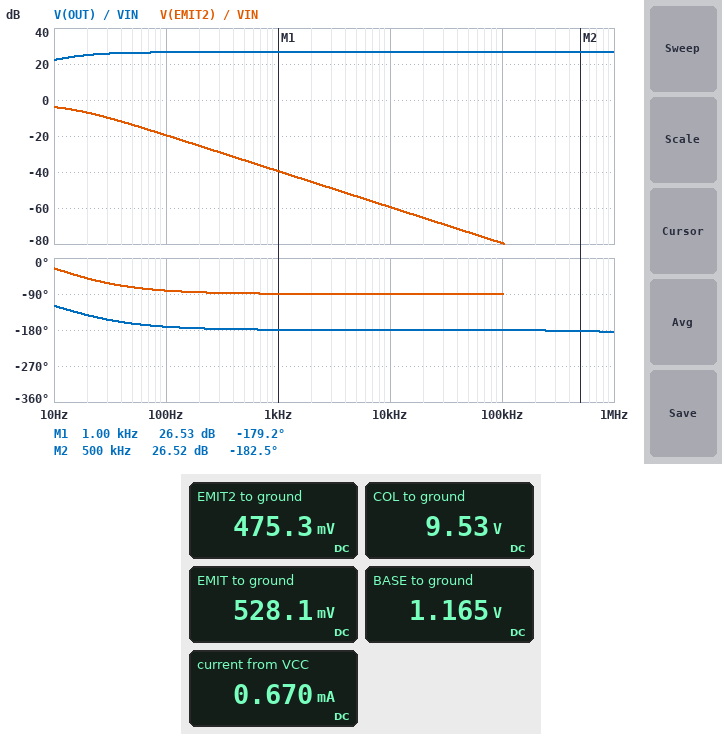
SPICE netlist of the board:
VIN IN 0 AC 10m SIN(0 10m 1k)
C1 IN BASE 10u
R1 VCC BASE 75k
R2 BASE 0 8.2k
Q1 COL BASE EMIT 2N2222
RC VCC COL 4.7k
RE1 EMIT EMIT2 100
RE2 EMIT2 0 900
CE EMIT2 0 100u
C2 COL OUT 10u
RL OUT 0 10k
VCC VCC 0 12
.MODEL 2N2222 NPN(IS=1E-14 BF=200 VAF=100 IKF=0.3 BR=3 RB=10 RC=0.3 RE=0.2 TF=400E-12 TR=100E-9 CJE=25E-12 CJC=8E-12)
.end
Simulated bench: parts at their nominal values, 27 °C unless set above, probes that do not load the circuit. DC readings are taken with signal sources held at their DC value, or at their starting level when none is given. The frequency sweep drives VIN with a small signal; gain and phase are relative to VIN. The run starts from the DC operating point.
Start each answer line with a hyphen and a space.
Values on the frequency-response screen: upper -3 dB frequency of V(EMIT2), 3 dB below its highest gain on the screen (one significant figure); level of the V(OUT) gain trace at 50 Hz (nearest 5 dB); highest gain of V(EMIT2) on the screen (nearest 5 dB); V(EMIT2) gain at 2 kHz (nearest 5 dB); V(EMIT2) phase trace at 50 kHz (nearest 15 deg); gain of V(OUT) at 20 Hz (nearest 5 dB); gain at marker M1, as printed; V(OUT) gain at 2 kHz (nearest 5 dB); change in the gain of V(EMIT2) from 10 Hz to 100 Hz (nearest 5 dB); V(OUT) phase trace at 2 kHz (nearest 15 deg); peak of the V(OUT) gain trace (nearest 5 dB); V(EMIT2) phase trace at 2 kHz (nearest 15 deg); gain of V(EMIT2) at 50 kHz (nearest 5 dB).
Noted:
- 20 Hz
- 25 dB
- -5 dB
- -45 dB
- -90 deg
- 25 dB
- 26.53 dB
- 25 dB
- -15 dB
- -180 deg
- 25 dB
- -90 deg
- -75 dB
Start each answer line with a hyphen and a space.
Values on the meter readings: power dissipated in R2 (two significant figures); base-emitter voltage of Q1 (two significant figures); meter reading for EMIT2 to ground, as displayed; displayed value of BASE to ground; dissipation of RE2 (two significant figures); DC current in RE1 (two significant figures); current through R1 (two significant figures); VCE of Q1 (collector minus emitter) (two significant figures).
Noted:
- 170 µW
- 640 mV
- 475.3 mV
- 1.165 V
- 250 µW
- 530 µA
- 140 µA
- 9.0 V
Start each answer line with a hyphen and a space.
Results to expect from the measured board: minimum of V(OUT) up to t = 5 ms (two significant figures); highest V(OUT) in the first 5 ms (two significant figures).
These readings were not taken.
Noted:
- -210 mV
- 210 mV
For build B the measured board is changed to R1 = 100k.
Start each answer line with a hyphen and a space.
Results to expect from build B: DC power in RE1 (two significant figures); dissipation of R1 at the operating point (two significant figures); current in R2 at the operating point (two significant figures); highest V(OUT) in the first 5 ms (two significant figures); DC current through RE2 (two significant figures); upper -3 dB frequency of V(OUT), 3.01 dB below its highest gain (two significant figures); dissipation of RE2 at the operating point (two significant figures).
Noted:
- 7.8 µW
- 1.2 mW
- 110 µA
- 160 mV
- 280 µA
- 14 MHz
- 71 µW
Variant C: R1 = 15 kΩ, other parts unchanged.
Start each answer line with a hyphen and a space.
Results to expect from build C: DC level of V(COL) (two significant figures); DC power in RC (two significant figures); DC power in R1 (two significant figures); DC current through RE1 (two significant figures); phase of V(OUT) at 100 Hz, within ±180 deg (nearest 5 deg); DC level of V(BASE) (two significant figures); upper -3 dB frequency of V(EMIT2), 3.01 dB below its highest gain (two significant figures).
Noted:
- 2.3 V
- 20 mW
- 5.4 mW
- 2.3 mA
- 15 deg
- 3.0 V
- 130 Hz
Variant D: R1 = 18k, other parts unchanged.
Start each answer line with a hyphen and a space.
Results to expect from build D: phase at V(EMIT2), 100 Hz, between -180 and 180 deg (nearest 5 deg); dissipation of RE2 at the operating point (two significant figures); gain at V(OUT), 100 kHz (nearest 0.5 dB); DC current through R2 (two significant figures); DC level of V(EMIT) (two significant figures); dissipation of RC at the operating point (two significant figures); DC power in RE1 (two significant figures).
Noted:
- -40 deg
- 4.4 mW
- -10.0 dB
- 350 µA
- 2.2 V
- 20 mW
- 490 µW
